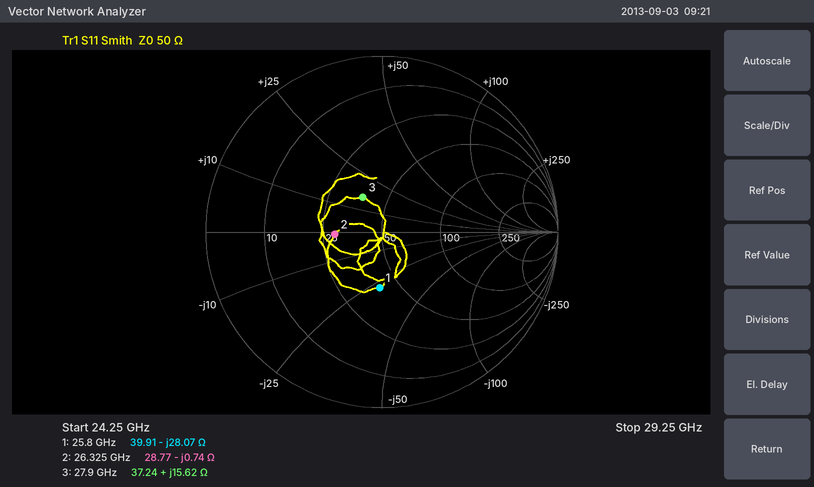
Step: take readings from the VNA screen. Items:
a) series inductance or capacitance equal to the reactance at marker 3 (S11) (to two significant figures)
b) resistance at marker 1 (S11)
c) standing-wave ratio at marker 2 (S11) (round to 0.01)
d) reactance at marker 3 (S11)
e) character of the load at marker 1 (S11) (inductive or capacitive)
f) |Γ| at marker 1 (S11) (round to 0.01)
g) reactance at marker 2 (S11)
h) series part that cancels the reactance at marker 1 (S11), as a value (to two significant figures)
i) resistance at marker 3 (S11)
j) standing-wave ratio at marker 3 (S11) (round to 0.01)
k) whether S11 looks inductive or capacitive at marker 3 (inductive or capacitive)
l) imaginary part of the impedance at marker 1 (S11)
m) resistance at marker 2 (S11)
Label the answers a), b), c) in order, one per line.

a) 89 pH
b) 39.91 Ω
c) 1.74
d) +15.62 Ω
e) capacitive
f) 0.32
g) -0.74 Ω
h) 170 pH
i) 37.24 Ω
j) 1.59
k) inductive
l) -28.07 Ω
m) 28.77 Ω
